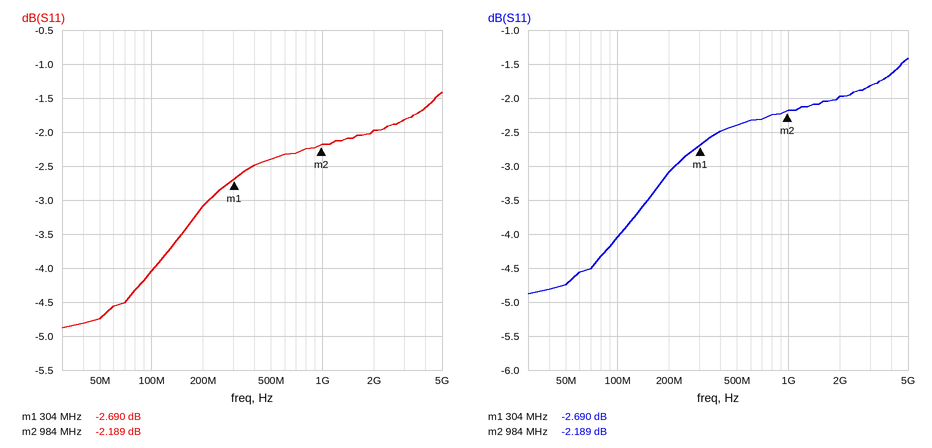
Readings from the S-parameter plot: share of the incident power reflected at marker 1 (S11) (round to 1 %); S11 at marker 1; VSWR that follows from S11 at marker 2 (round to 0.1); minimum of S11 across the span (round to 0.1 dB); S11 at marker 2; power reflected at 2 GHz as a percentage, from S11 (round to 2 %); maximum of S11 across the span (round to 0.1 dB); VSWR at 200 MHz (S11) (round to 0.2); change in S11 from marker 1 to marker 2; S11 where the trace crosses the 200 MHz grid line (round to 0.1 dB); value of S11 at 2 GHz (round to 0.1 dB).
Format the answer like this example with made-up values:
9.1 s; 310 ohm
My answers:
54 %; -2.690 dB; 8.0; -4.9 dB; -2.189 dB; 64 %; -1.4 dB; 5.6; 0.501 dB; -3.1 dB; -2.0 dB
